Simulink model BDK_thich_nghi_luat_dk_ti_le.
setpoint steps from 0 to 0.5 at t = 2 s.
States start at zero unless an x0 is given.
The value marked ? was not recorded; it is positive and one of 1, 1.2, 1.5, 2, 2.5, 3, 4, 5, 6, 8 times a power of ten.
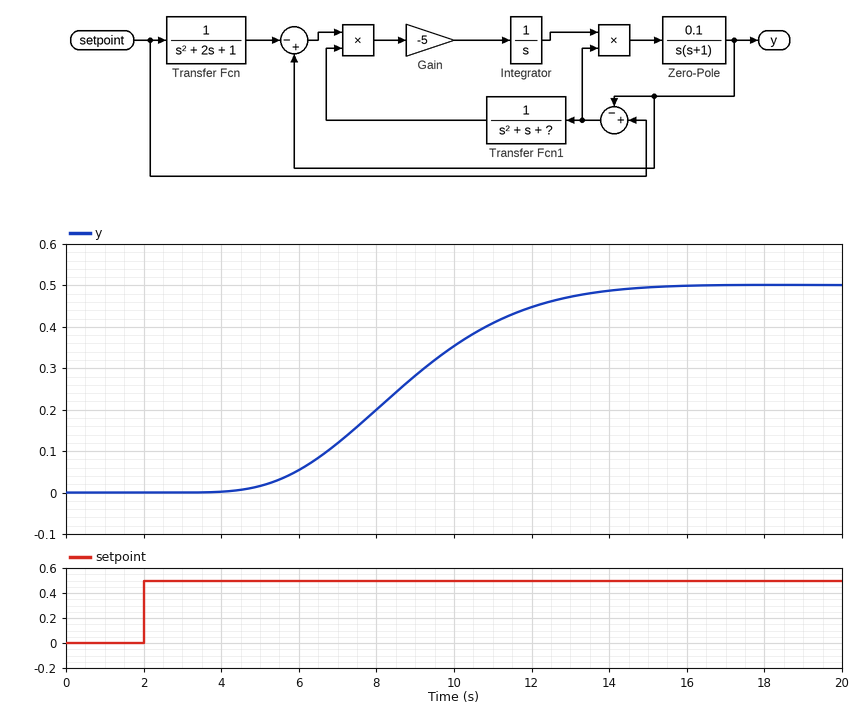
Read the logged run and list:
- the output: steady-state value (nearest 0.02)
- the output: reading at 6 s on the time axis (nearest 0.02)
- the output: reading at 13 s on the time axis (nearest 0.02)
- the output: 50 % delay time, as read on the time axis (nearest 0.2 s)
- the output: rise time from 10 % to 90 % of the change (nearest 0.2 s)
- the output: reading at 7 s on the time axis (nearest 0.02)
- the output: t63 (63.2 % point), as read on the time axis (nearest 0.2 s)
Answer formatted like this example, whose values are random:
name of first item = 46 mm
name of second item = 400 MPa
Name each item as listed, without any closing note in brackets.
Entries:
the output: steady-state value = 0.50
the output: reading at 6 s on the time axis = 0.06
the output: reading at 13 s on the time axis = 0.48
the output: 50 % delay time, as read on the time axis = 8.6 s
the output: rise time from 10 % to 90 % of the change = 6.2 s
the output: reading at 7 s on the time axis = 0.12
the output: t63 (63.2 % point), as read on the time axis = 9.4 s
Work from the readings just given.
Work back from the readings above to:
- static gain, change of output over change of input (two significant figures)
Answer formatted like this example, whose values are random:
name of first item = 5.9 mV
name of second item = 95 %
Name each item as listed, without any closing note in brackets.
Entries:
static gain, change of output over change of input = 1.0
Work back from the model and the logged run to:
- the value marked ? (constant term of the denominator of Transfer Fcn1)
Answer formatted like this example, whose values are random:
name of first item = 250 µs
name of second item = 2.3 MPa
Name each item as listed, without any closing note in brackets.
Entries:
the value marked ? = 1.5
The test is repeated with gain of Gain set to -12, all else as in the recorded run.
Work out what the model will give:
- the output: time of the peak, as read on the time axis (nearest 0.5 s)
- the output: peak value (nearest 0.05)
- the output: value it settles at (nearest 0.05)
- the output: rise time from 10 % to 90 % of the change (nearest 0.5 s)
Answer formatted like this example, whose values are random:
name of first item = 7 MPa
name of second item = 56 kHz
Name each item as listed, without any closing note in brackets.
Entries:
the output: time of the peak, as read on the time axis = 11.5 s
the output: peak value = 0.50
the output: value it settles at = 0.50
the output: rise time from 10 % to 90 % of the change = 3.5 s
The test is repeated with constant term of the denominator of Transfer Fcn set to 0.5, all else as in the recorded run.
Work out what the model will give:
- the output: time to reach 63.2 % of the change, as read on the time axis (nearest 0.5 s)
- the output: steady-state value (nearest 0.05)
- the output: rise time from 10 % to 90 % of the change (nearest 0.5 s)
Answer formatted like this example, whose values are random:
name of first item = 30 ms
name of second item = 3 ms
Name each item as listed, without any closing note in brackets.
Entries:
the output: time to reach 63.2 % of the change, as read on the time axis = 9.0 s
the output: steady-state value = 0.50
the output: rise time from 10 % to 90 % of the change = 5.0 s
